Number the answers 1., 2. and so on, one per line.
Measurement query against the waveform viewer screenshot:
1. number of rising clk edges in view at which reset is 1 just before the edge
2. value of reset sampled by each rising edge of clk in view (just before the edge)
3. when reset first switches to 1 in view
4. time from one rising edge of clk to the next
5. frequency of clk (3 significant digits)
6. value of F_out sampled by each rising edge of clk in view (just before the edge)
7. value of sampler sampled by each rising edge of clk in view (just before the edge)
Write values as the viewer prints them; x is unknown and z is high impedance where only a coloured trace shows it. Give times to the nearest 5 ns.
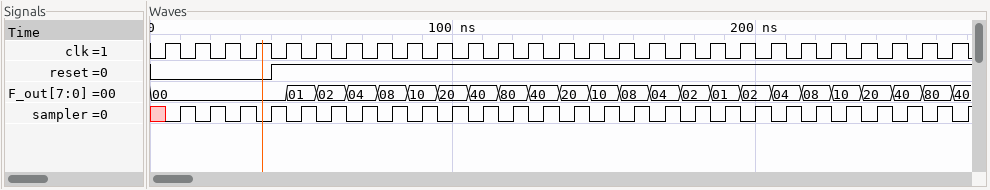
1. 23
2. 0 0 0 0 1 1 1 1 1 1 1 1 1 1 1 1 1 1 1 1 1 1 1 1 1 1 1
3. 40 ns
4. 10 ns
5. 100 MHz
6. 00, 00, 00, 00, 00, 01, 02, 04, 08, 10, 20, 40, 80, 40, 20, 10, 08, 04, 02, 01, 02, 04, 08, 10, 20, 40, 80
7. x 1 1 1 1 1 1 1 1 1 1 1 1 1 1 1 1 1 1 1 1 1 1 1 1 1 1
